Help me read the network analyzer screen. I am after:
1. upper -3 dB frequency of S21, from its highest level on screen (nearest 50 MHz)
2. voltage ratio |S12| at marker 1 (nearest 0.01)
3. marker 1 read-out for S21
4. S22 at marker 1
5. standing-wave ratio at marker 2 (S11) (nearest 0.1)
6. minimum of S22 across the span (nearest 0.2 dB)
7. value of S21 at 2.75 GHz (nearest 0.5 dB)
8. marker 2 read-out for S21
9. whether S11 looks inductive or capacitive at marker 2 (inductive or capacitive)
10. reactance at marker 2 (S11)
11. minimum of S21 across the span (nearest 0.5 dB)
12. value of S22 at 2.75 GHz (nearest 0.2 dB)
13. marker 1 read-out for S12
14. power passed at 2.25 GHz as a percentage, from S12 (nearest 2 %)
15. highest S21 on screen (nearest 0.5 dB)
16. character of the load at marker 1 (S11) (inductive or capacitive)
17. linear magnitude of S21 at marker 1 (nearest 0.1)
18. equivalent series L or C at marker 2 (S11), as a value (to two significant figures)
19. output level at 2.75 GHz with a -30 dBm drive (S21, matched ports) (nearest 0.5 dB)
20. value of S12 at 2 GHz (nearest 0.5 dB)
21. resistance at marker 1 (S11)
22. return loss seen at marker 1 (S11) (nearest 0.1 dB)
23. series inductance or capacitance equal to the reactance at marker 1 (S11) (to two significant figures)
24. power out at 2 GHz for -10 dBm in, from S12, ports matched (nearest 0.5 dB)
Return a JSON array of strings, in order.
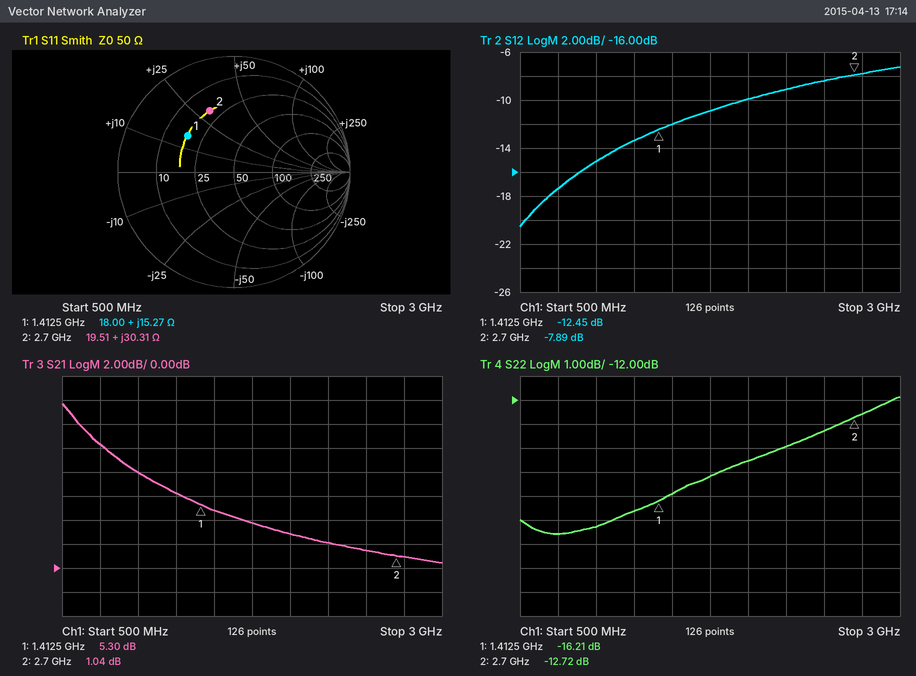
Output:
["700 MHz", "0.24", "5.30 dB", "-16.21 dB", "3.6", "-17.6 dB", "1.0 dB", "1.04 dB", "inductive", "+30.31 Ω", "0.5 dB", "-12.6 dB", "-12.45 dB", "12 %", "13.5 dB", "inductive", "1.8", "1.8 nH", "-29.0 dBm", "-10.0 dB", "18.00 Ω", "5.9 dB", "1.7 nH", "-20.0 dBm"]
